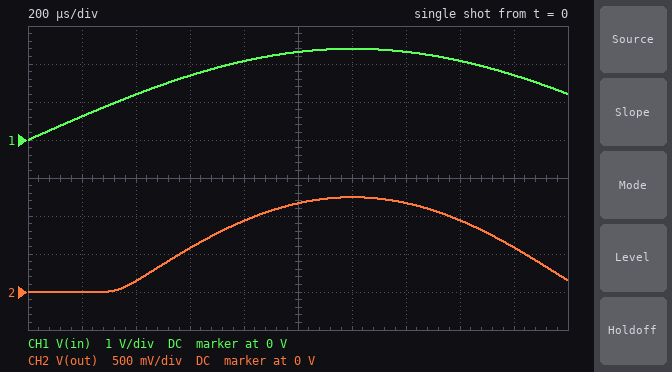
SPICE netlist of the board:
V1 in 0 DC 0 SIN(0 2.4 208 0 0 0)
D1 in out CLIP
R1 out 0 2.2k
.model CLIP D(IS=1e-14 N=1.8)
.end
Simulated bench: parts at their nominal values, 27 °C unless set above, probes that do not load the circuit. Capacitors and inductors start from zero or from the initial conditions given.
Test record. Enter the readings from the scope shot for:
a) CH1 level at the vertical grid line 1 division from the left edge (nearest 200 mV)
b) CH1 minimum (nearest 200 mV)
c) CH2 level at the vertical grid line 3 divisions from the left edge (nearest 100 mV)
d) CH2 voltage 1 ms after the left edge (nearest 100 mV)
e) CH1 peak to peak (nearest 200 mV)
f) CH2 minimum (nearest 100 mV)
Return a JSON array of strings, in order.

["600 mV", "0 V", "600 mV", "1.2 V", "2.4 V", "0 V"]
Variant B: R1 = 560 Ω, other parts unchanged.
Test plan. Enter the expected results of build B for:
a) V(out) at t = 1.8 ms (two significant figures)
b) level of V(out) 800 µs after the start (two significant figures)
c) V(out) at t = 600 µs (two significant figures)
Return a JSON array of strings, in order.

["530 mV", "880 mV", "520 mV"]
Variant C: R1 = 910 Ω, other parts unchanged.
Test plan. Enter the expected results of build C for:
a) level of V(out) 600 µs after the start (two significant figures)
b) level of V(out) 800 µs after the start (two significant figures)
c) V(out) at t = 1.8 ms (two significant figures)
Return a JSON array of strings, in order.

["540 mV", "900 mV", "550 mV"]
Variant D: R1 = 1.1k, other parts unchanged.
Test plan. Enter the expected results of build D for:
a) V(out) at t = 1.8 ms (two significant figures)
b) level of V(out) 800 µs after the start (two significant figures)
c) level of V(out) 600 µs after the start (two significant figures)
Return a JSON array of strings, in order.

["560 mV", "910 mV", "550 mV"]
